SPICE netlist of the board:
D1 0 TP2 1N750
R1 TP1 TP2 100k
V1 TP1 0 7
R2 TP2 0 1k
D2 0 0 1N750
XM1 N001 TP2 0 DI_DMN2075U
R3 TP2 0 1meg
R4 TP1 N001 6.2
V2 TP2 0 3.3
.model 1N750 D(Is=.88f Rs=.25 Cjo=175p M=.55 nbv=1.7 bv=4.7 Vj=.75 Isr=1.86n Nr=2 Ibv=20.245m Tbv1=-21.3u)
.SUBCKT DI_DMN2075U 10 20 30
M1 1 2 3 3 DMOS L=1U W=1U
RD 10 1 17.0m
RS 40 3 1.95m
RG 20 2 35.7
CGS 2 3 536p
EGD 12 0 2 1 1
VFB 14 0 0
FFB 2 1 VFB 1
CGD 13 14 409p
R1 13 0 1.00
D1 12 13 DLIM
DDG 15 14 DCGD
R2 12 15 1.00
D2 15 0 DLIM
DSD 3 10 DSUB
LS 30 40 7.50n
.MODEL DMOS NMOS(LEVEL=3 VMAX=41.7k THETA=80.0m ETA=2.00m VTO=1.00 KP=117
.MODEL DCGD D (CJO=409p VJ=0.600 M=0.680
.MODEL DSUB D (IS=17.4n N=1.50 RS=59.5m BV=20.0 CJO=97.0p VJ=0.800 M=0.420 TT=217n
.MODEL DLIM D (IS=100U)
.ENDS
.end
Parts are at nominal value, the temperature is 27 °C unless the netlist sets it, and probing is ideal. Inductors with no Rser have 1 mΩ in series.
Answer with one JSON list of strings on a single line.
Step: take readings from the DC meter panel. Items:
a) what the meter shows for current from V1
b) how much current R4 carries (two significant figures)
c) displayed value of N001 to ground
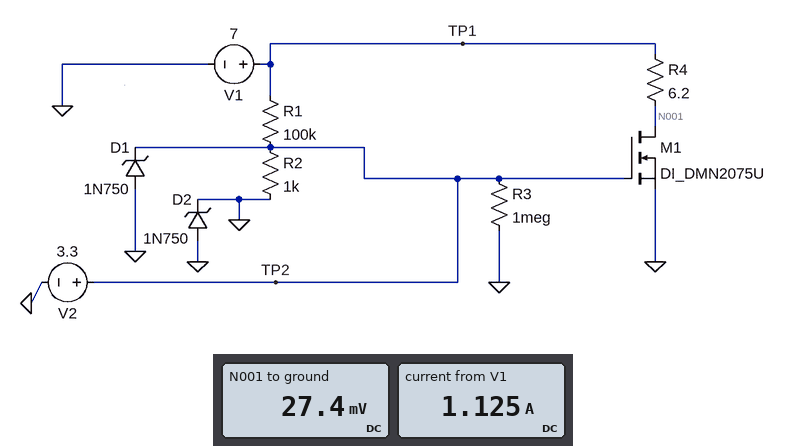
["1.125 A", "1.1 A", "27.4 mV"]
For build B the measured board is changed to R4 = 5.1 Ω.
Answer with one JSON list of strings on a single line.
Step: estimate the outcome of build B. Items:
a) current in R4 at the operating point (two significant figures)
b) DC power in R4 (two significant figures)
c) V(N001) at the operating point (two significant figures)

["1.4 A", "9.5 W", "33 mV"]
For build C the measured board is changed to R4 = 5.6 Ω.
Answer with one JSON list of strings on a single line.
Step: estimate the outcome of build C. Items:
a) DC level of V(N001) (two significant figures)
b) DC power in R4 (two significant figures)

["30 mV", "8.7 W"]
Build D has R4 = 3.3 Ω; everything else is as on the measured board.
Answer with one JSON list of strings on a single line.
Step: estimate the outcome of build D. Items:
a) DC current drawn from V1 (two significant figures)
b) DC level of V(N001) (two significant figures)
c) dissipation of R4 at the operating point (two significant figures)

["2.1 A", "51 mV", "15 W"]
